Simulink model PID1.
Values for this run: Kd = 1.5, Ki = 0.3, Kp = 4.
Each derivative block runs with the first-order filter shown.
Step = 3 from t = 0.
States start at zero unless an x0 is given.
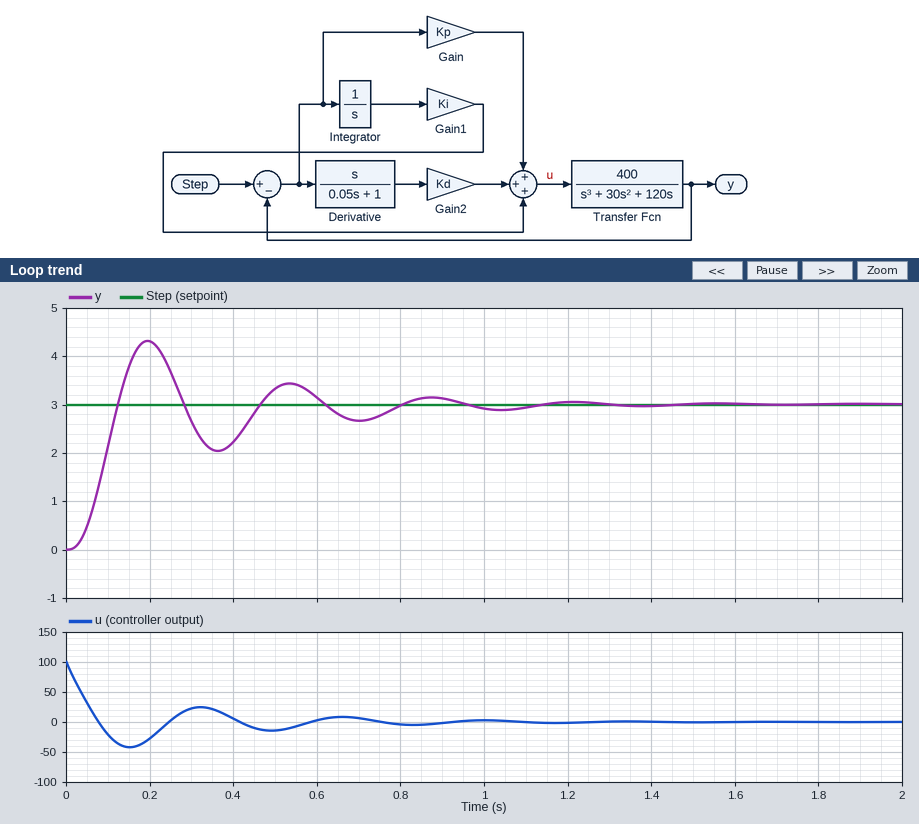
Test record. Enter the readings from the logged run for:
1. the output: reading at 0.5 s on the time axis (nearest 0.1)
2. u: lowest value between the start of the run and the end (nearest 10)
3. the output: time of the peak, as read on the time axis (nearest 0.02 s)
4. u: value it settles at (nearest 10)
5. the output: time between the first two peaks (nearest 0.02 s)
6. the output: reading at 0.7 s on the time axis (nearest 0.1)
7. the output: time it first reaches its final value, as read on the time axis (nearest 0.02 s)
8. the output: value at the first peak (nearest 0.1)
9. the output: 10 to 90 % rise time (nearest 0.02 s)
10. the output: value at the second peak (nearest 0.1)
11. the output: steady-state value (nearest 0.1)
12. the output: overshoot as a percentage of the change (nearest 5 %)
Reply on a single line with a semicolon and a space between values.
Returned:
3.3; -40; 0.20 s; 0; 0.34 s; 2.7; 0.12 s; 4.3; 0.08 s; 3.4; 3.0; 45 %
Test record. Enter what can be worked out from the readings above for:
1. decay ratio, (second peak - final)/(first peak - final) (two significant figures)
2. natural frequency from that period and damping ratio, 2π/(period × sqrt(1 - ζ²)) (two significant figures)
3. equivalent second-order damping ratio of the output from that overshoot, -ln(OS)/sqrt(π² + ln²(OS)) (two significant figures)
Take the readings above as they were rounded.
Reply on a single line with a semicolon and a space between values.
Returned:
0.31; 19 rad/s; 0.25
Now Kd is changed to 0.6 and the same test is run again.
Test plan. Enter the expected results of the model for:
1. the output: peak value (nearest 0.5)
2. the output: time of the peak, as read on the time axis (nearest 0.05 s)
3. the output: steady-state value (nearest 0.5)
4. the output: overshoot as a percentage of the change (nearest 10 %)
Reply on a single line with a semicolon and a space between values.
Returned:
4.0; 0.30 s; 3.0; 30 %
